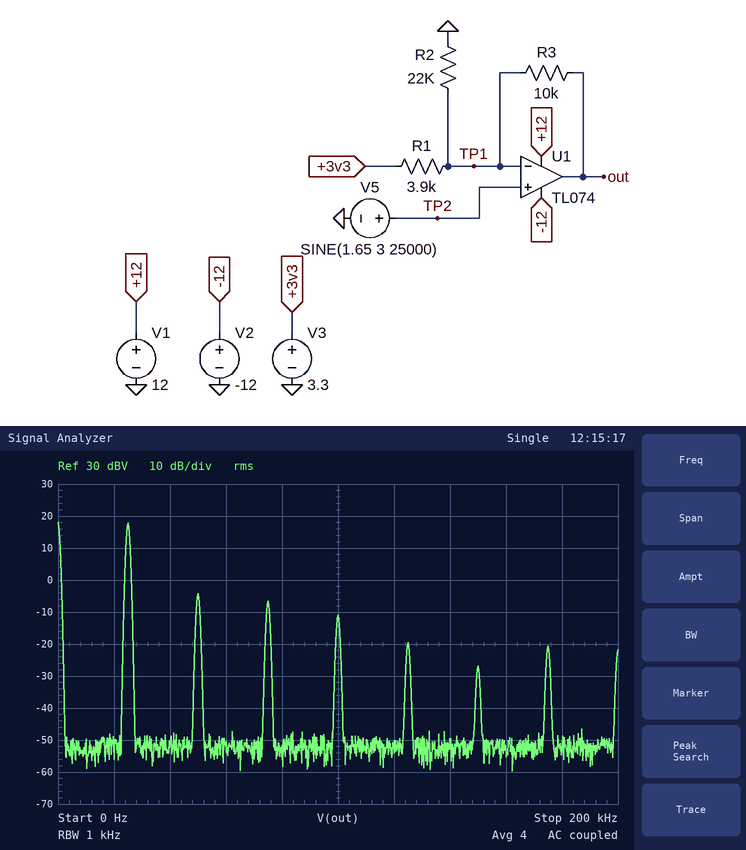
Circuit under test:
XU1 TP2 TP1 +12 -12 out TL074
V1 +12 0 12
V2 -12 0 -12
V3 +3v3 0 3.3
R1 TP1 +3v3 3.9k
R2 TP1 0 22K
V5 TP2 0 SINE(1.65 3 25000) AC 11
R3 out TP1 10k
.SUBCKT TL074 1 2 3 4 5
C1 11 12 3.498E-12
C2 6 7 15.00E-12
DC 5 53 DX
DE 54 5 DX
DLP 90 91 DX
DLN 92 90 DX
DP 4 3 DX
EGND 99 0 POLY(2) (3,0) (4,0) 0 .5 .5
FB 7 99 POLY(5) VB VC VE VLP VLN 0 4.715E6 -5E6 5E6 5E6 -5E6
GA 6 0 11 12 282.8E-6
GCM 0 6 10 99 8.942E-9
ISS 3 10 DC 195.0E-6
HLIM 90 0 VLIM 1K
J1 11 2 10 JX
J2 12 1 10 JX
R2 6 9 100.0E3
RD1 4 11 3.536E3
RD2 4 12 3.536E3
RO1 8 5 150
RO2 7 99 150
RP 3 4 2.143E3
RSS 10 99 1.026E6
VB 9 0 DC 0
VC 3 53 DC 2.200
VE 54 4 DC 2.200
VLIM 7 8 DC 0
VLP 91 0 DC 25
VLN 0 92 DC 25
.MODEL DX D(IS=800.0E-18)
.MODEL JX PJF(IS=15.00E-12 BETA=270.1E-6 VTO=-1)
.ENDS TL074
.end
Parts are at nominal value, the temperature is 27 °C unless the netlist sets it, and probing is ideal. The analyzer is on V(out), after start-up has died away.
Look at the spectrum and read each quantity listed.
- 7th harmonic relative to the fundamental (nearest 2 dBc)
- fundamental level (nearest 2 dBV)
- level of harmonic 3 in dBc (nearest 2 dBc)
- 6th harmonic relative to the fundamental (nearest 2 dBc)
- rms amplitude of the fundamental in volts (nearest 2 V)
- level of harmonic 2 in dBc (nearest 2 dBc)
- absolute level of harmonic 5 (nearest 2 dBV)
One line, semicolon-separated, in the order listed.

-38 dBc; 18 dBV; -24 dBc; -44 dBc; 8 V; -22 dBc; -20 dBV
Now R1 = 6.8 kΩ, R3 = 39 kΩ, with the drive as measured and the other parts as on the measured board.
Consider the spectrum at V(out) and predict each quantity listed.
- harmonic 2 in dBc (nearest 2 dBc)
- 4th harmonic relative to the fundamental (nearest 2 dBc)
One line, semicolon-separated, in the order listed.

-14 dBc; -18 dBc
